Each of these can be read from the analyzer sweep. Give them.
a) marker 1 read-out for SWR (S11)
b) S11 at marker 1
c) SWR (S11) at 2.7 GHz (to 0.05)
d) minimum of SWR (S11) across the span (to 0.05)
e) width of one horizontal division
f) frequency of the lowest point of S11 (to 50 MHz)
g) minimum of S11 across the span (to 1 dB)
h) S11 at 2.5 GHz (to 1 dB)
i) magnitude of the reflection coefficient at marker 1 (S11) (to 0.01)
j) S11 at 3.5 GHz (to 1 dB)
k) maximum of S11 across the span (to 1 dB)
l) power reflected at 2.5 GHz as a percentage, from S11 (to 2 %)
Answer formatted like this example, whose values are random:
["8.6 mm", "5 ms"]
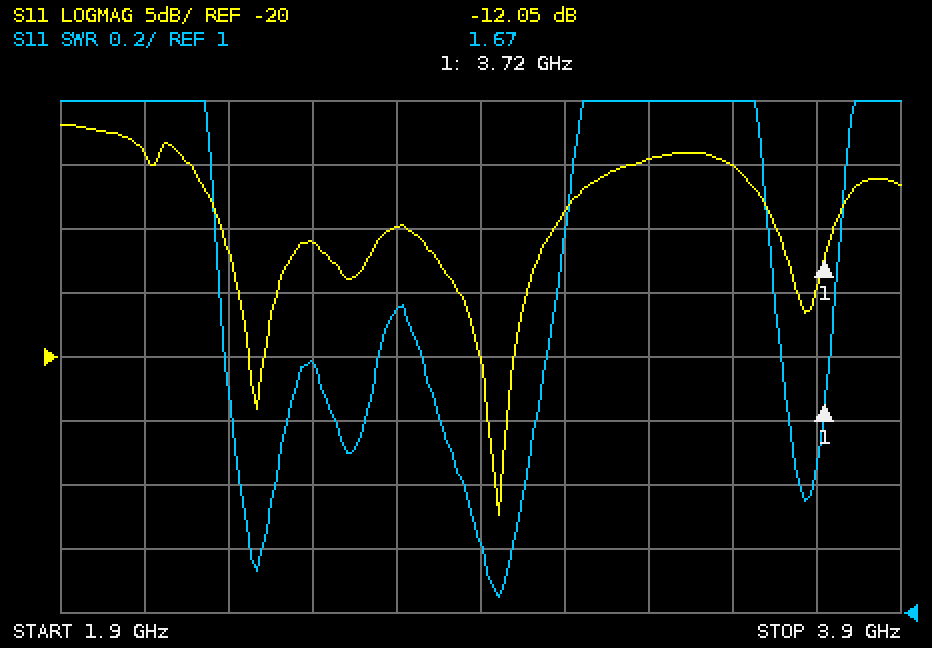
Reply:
["1.67", "-12.05 dB", "1.95", "1.05", "200 MHz", "2.95 GHz", "-32 dB", "-11 dB", "0.25", "-5 dB", "-2 dB", "8 %"]
